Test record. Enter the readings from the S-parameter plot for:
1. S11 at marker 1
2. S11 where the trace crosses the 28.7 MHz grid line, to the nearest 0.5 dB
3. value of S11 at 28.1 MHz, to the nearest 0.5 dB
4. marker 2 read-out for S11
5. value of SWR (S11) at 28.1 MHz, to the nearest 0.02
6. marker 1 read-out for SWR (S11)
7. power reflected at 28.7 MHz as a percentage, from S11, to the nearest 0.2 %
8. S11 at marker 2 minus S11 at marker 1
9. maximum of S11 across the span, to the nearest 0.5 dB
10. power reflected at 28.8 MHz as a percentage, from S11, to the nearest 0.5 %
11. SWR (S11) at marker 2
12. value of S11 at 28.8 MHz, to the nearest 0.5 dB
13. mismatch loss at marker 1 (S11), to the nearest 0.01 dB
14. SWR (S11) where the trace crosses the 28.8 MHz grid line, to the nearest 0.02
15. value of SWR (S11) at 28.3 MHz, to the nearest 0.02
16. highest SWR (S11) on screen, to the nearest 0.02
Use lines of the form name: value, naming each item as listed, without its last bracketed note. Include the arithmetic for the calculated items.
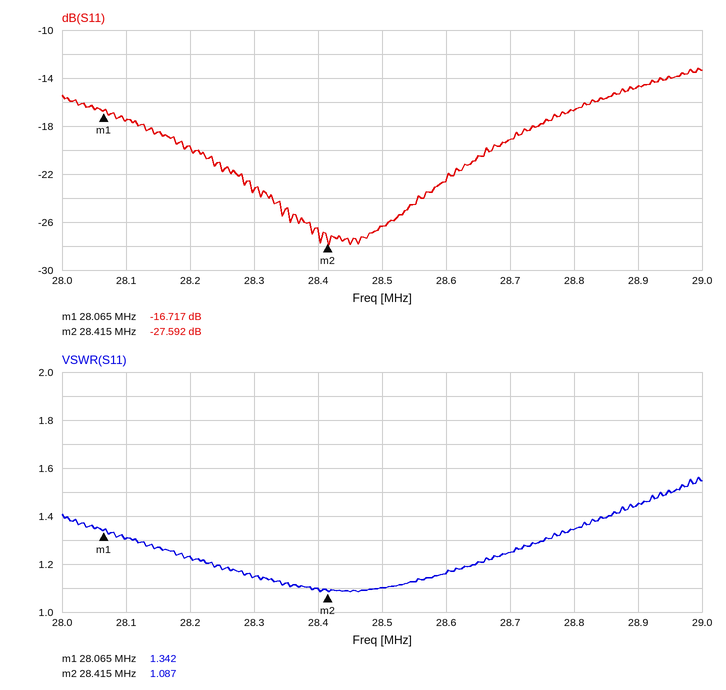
S11 at marker 1: -16.717 dB
S11 where the trace crosses the 28.7 MHz grid line, to the nearest 0.5 dB: -19.0 dB
value of S11 at 28.1 MHz, to the nearest 0.5 dB: -17.5 dB
marker 2 read-out for S11: -27.592 dB
value of SWR (S11) at 28.1 MHz, to the nearest 0.02: 1.30
marker 1 read-out for SWR: 1.342
power reflected at 28.7 MHz as a percentage, from S11, to the nearest 0.2 %: 10^(-19/10) ≈ 1.26 %, so 1.2 % to the nearest 0.2 %
S11 at marker 2 minus S11 at marker 1: -27.592 − (-16.717) = -10.875 dB
maximum of S11 across the span, to the nearest 0.5 dB: -13.0 dB
power reflected at 28.8 MHz as a percentage, from S11, to the nearest 0.5 %: 10^(-16.5/10) ≈ 2.24 %, so 2.0 % to the nearest 0.5 %
SWR (S11) at marker 2: 1.087
value of S11 at 28.8 MHz, to the nearest 0.5 dB: -16.5 dB
mismatch loss at marker 1 (S11), to the nearest 0.01 dB: −10 log10(1 − 10^(-16.717/10)) ≈ 0.09 dB
SWR (S11) where the trace crosses the 28.8 MHz grid line, to the nearest 0.02: 1.34
value of SWR (S11) at 28.3 MHz, to the nearest 0.02: 1.14
highest SWR (S11) on screen, to the nearest 0.02: 1.56
